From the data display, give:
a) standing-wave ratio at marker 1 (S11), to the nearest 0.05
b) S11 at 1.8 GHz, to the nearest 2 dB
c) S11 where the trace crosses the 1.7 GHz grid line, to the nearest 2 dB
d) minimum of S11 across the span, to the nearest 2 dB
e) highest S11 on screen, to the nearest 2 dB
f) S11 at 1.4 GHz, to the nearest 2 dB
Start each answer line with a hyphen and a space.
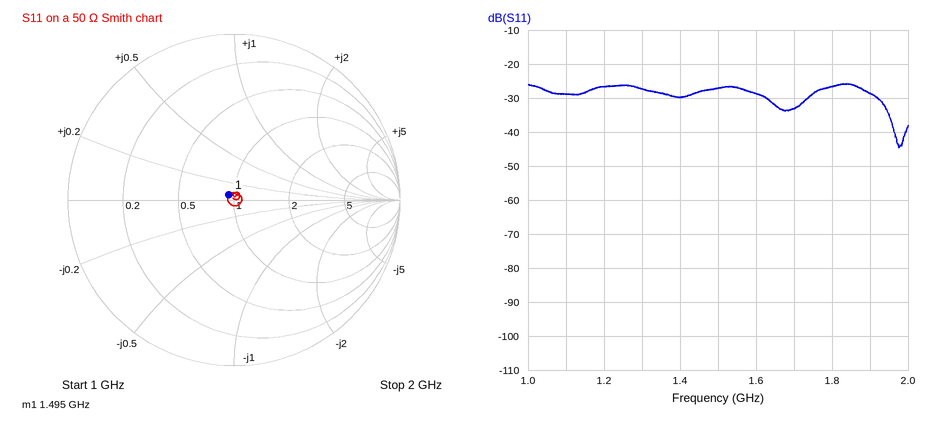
- 1.10
- -26 dB
- -34 dB
- -44 dB
- -26 dB
- -30 dB
